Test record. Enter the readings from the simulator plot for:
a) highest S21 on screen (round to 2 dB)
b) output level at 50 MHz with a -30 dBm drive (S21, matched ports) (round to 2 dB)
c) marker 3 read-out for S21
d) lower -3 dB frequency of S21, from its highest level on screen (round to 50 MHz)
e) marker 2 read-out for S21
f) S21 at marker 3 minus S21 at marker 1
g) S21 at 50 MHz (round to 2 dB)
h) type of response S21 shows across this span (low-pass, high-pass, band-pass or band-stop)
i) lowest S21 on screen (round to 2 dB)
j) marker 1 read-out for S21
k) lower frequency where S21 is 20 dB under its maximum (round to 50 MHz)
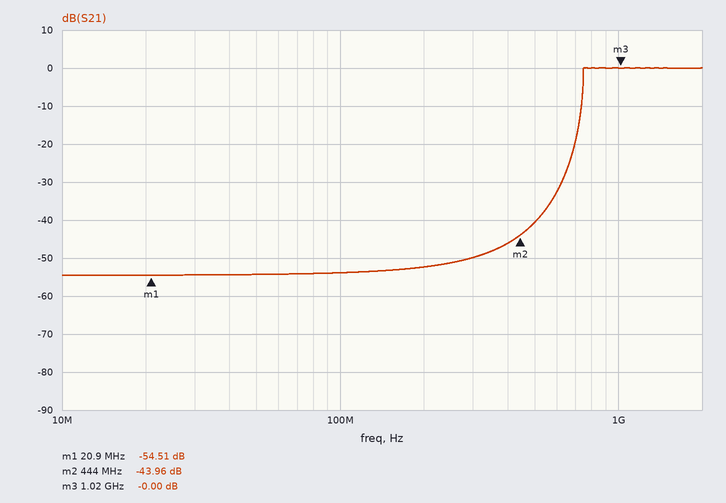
0 dB
-84 dBm
-0.00 dB
750 MHz
-43.96 dB
54.51 dB
-54 dB
high-pass
-54 dB
-54.51 dB
700 MHz
